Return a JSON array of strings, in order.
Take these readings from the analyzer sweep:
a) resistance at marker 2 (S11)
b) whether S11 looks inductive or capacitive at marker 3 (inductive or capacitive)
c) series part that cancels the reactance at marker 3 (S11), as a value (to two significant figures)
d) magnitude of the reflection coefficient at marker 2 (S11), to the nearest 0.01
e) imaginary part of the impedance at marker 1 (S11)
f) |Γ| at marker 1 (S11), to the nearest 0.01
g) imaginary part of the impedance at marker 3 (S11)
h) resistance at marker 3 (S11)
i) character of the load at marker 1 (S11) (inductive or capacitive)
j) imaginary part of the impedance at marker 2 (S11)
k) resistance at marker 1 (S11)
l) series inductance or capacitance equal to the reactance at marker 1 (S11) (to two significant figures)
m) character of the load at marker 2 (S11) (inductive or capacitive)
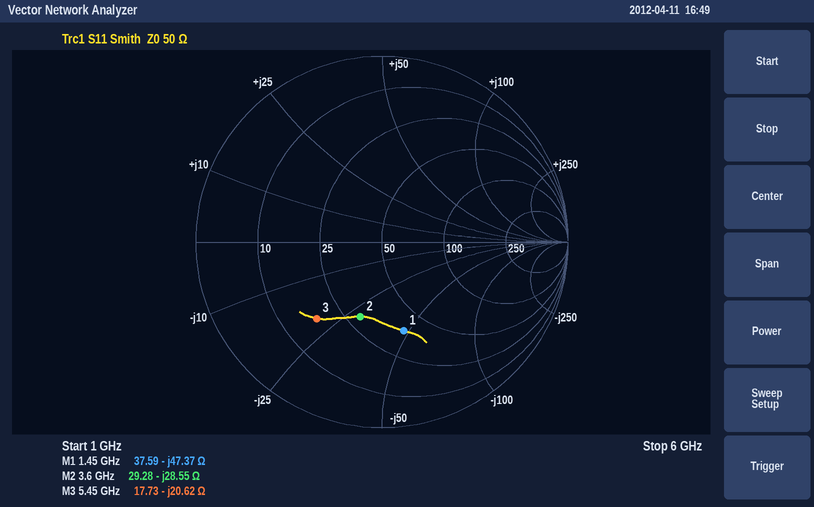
["29.28 Ω", "capacitive", "600 pH", "0.42", "-47.37 Ω", "0.49", "-20.62 Ω", "17.73 Ω", "capacitive", "-28.55 Ω", "37.59 Ω", "2.3 pF", "capacitive"]
